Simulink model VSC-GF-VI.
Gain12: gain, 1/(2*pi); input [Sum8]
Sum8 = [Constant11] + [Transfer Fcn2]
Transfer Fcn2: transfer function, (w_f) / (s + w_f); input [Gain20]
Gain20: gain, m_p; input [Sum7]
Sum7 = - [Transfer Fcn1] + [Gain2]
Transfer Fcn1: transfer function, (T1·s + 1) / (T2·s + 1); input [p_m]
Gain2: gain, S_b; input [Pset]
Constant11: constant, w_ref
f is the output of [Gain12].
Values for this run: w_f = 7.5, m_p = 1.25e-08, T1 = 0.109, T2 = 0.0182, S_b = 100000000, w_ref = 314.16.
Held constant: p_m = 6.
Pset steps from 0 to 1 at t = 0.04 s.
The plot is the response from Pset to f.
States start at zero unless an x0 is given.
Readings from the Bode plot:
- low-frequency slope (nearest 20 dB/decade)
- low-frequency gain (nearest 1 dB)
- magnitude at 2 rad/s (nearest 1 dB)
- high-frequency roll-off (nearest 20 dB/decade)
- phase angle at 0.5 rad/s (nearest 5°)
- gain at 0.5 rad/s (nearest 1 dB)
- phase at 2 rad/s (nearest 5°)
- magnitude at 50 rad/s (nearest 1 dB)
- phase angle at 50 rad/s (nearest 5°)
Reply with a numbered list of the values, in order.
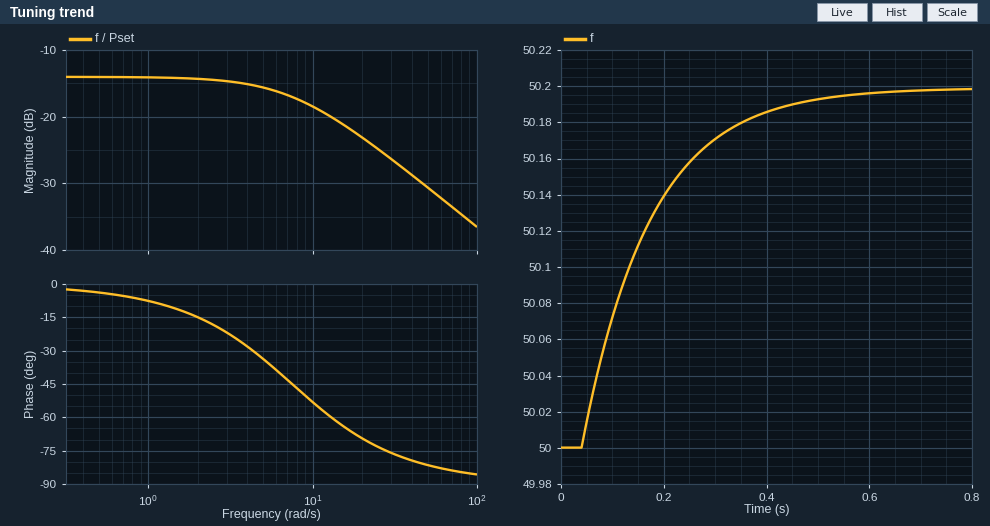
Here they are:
1. 0 dB/decade
2. -14 dB
3. -14 dB
4. -20 dB/decade
5. -5°
6. -14 dB
7. -15°
8. -31 dB
9. -80°
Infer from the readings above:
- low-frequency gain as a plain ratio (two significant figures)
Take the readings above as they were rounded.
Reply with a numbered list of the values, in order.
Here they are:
1. 0.20
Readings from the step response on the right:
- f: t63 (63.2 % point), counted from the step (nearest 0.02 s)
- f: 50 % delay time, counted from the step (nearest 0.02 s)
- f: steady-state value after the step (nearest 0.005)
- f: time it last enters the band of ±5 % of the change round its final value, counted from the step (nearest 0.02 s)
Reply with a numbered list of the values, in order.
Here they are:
1. 0.14 s
2. 0.10 s
3. 50.200
4. 0.40 s
